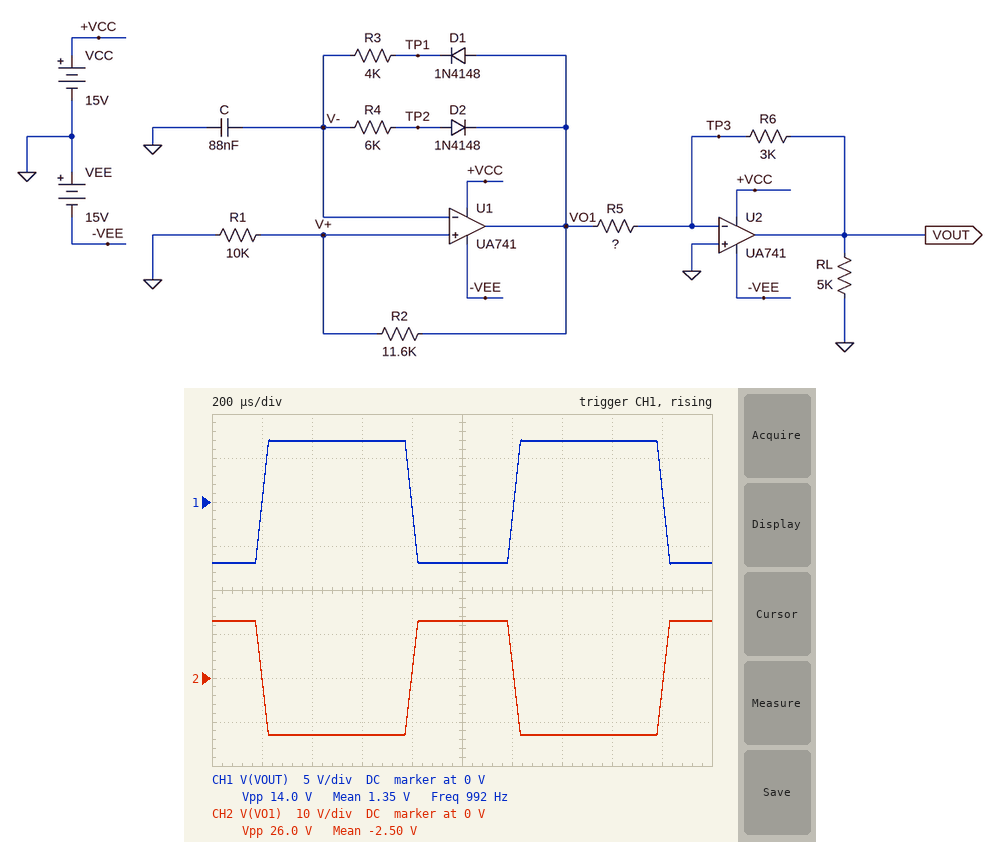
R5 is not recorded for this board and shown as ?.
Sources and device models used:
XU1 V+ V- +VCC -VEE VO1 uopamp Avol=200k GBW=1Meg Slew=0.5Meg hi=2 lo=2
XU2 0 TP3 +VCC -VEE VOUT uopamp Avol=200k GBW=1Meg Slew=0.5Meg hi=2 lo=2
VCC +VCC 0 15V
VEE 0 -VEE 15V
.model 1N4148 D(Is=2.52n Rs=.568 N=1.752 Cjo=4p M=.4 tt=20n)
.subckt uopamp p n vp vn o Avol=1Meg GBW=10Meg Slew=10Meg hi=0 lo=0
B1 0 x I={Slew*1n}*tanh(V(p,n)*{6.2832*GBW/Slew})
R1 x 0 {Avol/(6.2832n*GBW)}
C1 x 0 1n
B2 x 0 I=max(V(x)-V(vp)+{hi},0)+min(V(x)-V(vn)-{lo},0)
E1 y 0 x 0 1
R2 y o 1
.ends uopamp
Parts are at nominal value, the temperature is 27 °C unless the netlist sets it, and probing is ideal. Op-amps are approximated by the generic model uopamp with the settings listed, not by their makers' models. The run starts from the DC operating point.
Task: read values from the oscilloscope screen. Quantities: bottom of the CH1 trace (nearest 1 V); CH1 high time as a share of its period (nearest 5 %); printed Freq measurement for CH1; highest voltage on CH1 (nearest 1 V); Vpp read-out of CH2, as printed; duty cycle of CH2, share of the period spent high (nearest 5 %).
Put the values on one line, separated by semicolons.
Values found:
-7 V; 60 %; 992 Hz; 7 V; 26.0 V; 40 %
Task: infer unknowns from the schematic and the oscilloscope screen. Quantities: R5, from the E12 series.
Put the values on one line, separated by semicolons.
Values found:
5.6 kΩ
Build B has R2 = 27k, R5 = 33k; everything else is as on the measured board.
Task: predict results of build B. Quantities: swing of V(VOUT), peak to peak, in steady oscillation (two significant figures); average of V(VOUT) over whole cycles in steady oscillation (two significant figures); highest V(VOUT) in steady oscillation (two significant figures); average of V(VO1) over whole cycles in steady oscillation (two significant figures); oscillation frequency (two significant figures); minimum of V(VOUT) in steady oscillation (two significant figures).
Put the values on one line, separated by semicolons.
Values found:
2.4 V; 210 mV; 1.2 V; -2.3 V; 1.7 kHz; -1.2 V
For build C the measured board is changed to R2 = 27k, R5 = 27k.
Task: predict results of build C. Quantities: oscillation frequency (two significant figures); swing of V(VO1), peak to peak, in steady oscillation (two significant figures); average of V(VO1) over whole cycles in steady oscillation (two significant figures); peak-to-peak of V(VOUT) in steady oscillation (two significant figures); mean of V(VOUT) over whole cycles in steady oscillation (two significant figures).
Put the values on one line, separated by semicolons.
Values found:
1.7 kHz; 26 V; -2.3 V; 2.9 V; 260 mV
